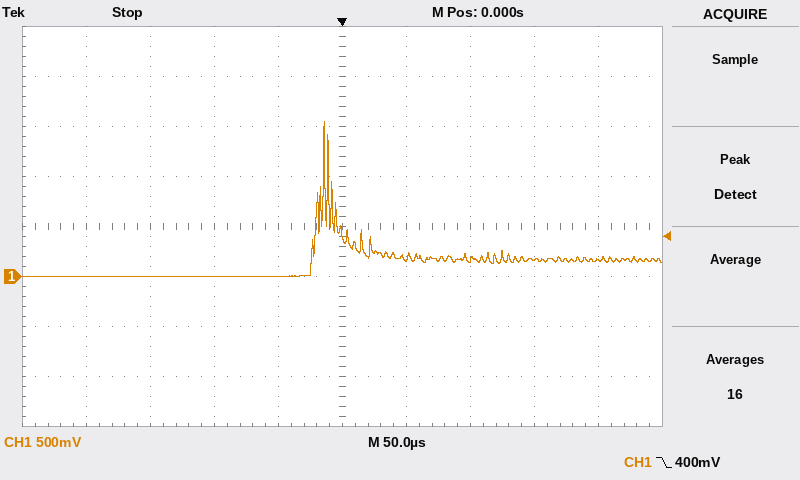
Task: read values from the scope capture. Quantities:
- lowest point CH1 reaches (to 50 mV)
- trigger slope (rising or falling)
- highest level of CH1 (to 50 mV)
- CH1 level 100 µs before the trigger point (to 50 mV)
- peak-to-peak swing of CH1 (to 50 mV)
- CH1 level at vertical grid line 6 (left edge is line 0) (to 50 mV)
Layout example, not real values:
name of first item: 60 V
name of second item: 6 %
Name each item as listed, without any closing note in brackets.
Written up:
lowest point CH1 reaches: 0 mV
trigger slope: falling
highest level of CH1: 1.55 V
CH1 level 100 µs before the trigger point: 0 mV
peak-to-peak swing of CH1: 1.55 V
CH1 level at vertical grid line 6 (left edge is line 0): 200 mV
